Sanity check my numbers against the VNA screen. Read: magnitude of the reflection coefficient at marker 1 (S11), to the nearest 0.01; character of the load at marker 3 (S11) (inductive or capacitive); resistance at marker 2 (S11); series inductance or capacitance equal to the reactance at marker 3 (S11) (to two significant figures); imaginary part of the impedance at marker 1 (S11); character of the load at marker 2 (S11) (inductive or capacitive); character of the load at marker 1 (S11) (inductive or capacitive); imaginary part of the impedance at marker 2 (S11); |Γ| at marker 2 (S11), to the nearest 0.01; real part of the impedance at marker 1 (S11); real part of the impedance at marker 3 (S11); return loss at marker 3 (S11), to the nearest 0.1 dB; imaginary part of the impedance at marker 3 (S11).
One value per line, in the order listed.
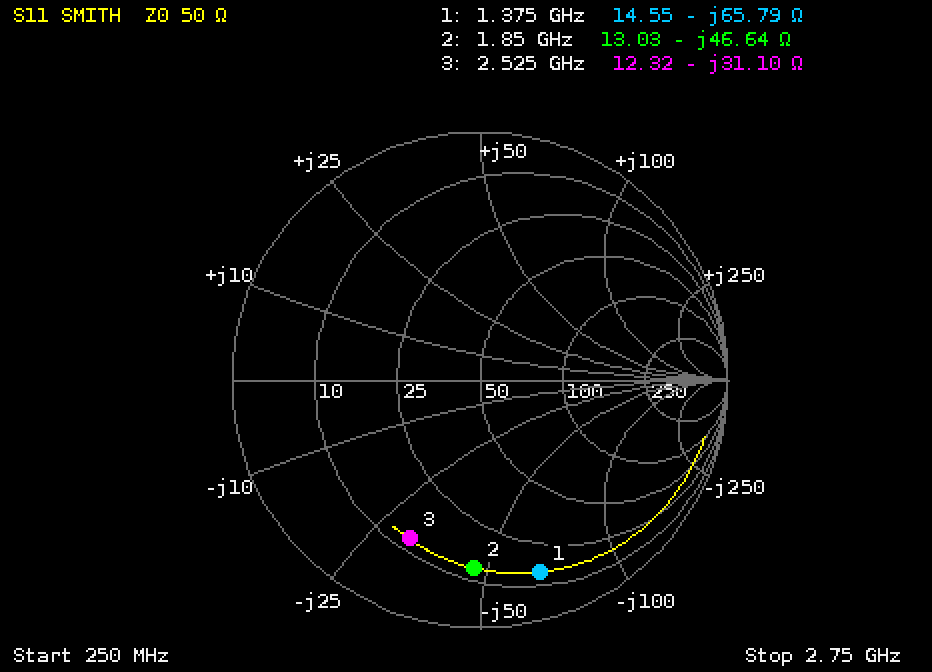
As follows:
0.81
capacitive
13.03 Ω
2.0 pF
-65.79 Ω
capacitive
capacitive
-46.64 Ω
0.76
14.55 Ω
12.32 Ω
3.1 dB
-31.10 Ω
